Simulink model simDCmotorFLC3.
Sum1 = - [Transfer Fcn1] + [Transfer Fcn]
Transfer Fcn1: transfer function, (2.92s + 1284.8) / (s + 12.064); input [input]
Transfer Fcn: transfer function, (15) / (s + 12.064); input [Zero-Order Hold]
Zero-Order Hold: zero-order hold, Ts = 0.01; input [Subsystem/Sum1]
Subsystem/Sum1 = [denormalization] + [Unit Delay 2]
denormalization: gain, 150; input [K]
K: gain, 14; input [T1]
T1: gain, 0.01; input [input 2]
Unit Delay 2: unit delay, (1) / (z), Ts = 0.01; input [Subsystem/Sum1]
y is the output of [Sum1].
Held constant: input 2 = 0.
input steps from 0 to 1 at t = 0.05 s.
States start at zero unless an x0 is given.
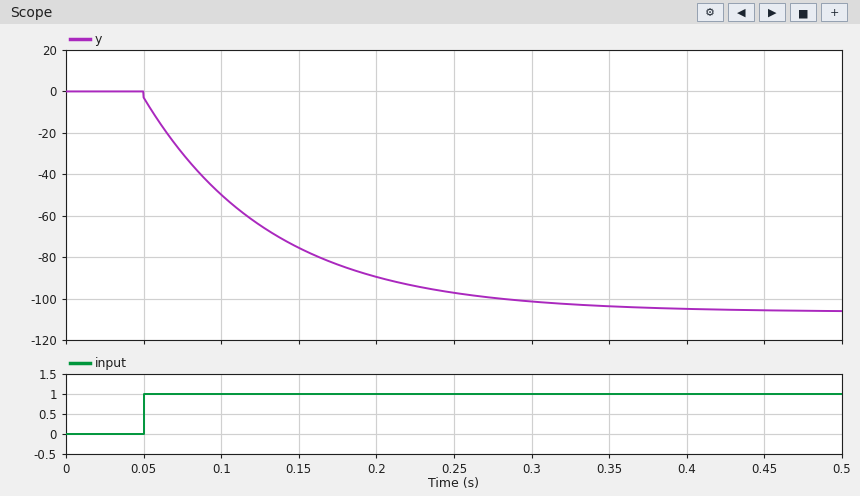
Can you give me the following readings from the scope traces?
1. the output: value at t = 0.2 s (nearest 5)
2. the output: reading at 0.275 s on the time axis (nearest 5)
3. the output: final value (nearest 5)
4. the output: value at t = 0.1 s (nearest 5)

-90
-100
-105
-50
